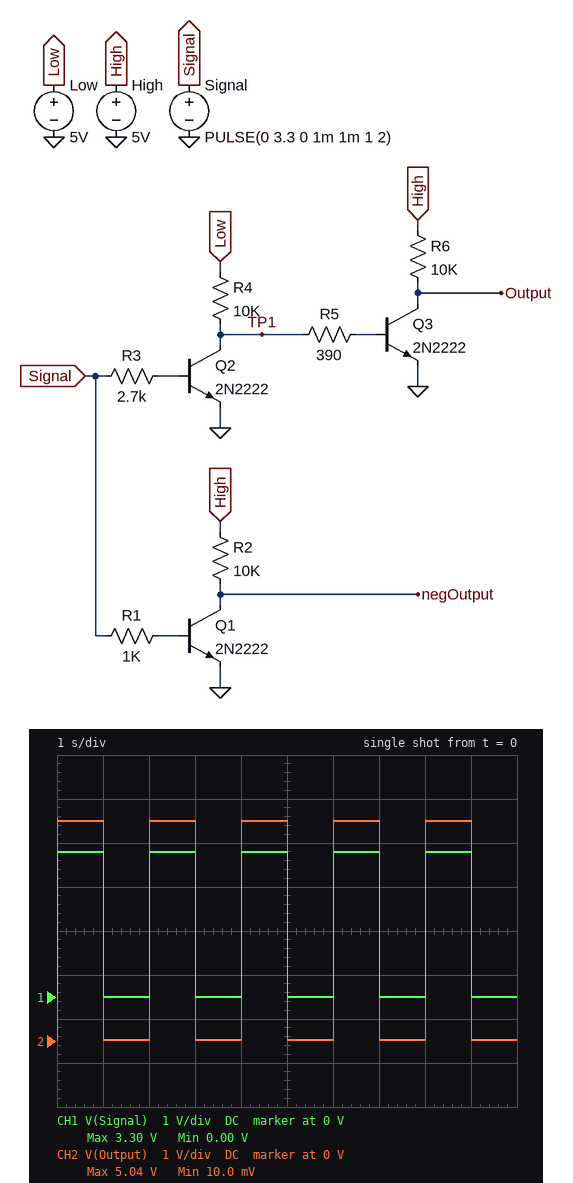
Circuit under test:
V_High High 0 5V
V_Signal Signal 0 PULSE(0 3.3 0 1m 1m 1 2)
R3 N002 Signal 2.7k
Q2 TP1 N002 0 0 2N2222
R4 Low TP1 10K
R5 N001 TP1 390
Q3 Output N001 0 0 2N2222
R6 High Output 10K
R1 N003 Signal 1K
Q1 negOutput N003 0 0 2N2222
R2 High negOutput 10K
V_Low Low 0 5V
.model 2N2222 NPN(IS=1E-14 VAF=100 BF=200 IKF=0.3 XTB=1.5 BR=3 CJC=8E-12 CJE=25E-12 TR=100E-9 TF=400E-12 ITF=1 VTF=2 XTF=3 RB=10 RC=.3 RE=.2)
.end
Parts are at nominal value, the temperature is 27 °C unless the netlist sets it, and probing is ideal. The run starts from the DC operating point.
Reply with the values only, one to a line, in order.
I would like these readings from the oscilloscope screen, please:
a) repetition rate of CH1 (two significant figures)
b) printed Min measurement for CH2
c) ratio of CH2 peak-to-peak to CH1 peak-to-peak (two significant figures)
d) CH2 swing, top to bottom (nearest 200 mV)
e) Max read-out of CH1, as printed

500 mHz
10.0 mV
1.5
5.0 V
3.30 V
